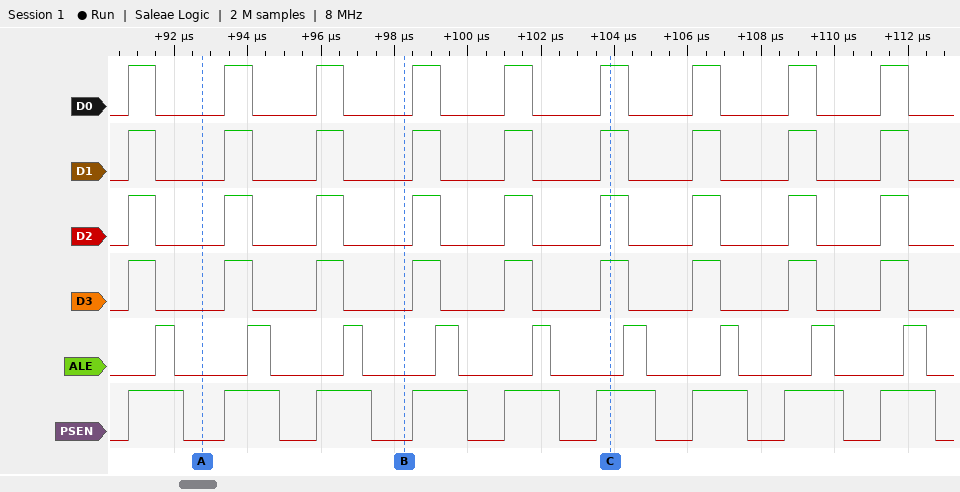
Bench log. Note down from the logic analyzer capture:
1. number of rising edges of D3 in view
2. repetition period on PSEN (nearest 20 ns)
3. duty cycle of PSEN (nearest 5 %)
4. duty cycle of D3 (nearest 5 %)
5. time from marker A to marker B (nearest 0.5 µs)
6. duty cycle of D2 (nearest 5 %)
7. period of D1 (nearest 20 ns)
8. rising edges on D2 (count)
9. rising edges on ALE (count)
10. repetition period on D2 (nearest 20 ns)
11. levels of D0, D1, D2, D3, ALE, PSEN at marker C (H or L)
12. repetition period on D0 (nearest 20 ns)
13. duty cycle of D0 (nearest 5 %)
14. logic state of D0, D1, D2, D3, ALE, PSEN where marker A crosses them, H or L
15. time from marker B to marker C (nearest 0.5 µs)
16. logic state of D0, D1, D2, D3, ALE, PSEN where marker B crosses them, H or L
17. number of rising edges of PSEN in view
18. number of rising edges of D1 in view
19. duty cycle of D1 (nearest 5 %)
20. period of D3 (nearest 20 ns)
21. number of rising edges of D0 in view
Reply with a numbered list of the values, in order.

1. 9
2. 2560 ns
3. 60 %
4. 30 %
5. 5.5 µs
6. 30 %
7. 2560 ns
8. 9
9. 9
10. 2560 ns
11. D0=H, D1=H, D2=H, D3=H, ALE=L, PSEN=H
12. 2560 ns
13. 30 %
14. D0=L, D1=L, D2=L, D3=L, ALE=L, PSEN=L
15. 5.5 µs
16. D0=L, D1=L, D2=L, D3=L, ALE=L, PSEN=L
17. 9
18. 9
19. 30 %
20. 2560 ns
21. 9
